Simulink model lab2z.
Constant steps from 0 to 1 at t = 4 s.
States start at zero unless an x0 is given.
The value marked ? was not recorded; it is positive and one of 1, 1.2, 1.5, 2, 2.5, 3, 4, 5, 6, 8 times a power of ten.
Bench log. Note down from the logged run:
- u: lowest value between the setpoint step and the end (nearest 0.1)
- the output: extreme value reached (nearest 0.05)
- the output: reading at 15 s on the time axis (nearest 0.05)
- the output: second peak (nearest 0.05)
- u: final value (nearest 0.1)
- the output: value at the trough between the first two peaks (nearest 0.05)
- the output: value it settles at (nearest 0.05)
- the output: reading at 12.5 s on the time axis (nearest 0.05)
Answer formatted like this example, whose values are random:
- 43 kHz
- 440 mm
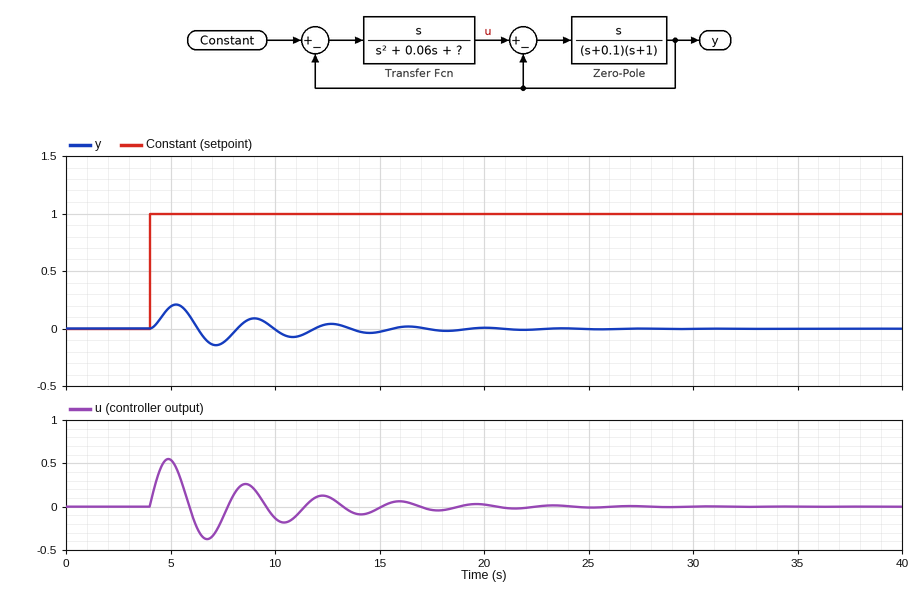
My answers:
- -0.4
- 0.20
- -0.05
- 0.10
- 0.0
- -0.15
- 0.00
- 0.05
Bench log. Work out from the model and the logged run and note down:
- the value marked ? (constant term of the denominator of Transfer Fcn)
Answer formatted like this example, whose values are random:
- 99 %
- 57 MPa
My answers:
- 2.5
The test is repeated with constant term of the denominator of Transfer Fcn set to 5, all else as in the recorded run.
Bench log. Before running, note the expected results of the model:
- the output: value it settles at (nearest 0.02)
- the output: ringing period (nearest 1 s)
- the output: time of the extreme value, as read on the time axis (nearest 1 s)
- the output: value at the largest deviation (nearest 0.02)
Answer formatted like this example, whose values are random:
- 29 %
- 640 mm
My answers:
- 0.00
- 3 s
- 5 s
- 0.14
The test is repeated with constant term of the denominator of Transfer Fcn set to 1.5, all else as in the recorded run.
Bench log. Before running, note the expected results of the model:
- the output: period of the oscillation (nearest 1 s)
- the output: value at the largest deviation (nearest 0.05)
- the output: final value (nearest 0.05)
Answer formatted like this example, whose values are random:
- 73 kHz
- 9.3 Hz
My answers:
- 5 s
- 0.25
- 0.00
